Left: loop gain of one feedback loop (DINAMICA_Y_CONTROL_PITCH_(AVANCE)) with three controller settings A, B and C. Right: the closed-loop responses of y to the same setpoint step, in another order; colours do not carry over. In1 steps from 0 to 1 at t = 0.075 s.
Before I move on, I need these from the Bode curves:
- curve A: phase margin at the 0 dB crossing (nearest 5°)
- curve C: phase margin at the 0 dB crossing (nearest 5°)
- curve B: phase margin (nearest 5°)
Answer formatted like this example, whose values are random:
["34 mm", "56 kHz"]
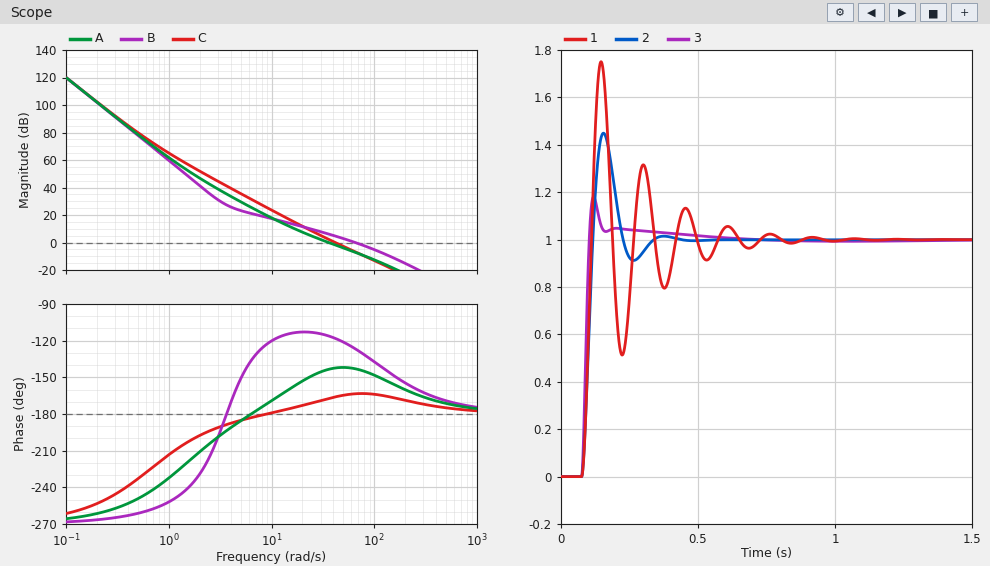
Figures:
["35°", "15°", "55°"]
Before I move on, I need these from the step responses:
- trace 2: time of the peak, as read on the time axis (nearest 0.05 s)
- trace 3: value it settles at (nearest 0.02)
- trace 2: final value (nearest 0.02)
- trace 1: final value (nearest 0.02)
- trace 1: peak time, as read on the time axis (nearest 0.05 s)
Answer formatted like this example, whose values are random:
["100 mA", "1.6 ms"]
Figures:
["0.15 s", "1.00", "1.00", "1.00", "0.15 s"]
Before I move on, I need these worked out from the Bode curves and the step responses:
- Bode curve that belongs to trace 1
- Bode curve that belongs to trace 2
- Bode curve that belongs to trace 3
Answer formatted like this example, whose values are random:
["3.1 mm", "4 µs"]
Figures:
["C", "A", "B"]
